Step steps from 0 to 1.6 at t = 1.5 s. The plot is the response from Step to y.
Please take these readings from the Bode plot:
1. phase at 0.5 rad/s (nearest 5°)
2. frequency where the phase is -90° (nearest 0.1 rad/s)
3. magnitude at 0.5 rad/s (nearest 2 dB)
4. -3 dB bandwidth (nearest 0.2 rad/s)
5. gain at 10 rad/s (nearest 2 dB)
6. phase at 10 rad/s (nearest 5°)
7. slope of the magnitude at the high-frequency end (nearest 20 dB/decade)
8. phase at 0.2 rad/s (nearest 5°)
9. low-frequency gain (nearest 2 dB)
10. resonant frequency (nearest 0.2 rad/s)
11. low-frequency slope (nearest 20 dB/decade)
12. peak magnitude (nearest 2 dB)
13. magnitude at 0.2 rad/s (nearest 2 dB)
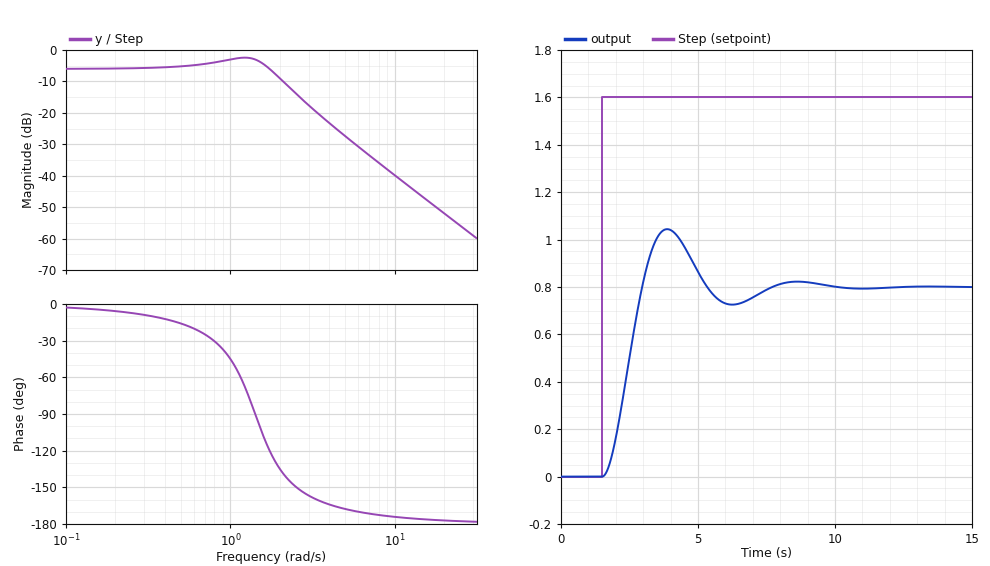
-15°
1.4 rad/s
-6 dB
2.0 rad/s
-40 dB
-175°
-40 dB/decade
-5°
-6 dB
1.2 rad/s
0 dB/decade
-2 dB
-6 dB
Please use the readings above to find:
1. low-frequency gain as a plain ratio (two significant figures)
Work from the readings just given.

0.50
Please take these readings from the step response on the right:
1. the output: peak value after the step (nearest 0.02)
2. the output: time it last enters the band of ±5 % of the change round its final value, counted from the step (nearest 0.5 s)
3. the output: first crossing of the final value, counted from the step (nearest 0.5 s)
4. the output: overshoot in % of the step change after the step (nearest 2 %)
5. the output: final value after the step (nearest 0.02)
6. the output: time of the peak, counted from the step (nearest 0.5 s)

1.04
5.5 s
1.5 s
30 %
0.80
2.5 s
